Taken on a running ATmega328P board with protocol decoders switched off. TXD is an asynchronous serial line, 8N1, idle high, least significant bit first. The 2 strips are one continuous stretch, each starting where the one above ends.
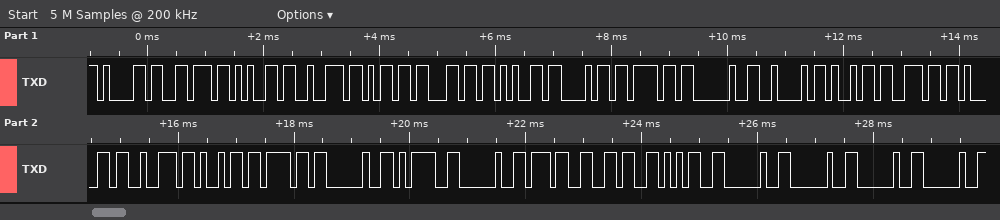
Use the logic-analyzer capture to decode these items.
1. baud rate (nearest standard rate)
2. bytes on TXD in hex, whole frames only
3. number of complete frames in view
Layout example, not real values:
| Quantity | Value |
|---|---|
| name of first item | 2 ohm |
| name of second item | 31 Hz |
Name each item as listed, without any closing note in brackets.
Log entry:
| Quantity | Value |
|---|---|
| baud rate | 9600 baud |
| bytes on TXD in hex, whole frames only | 61 76 65 72 6D 6C 65 68 6F 20 42 69 6E 61 72 69 6F 20 3D 20 37 36 35 20 20 20 20 |
| number of complete frames in view | 27 |
